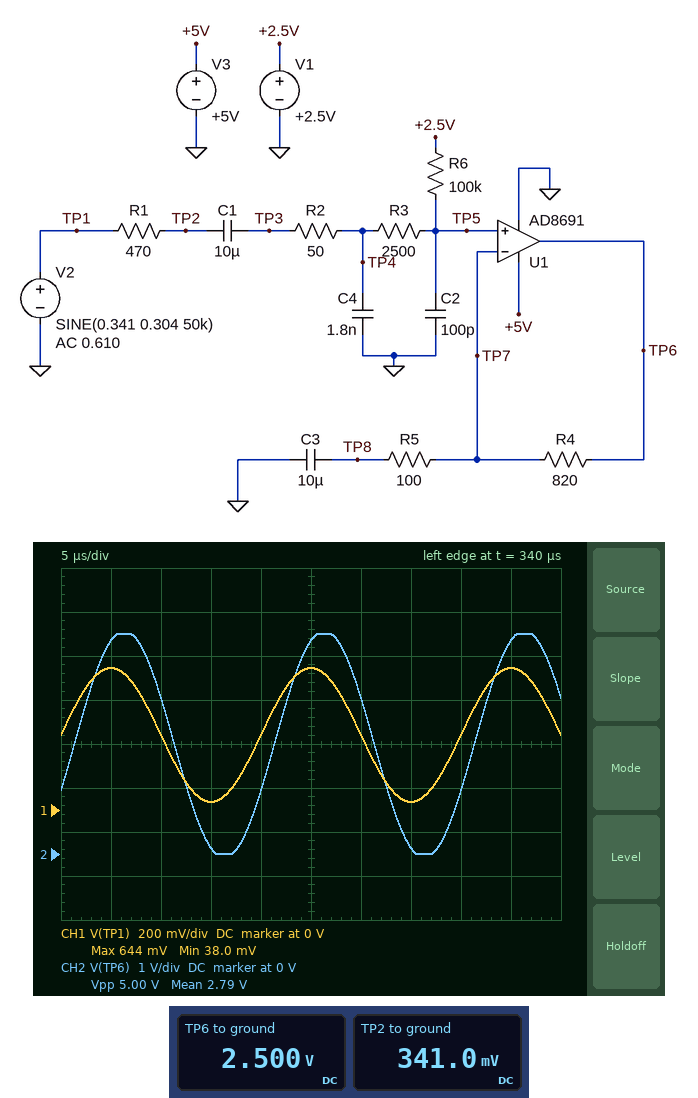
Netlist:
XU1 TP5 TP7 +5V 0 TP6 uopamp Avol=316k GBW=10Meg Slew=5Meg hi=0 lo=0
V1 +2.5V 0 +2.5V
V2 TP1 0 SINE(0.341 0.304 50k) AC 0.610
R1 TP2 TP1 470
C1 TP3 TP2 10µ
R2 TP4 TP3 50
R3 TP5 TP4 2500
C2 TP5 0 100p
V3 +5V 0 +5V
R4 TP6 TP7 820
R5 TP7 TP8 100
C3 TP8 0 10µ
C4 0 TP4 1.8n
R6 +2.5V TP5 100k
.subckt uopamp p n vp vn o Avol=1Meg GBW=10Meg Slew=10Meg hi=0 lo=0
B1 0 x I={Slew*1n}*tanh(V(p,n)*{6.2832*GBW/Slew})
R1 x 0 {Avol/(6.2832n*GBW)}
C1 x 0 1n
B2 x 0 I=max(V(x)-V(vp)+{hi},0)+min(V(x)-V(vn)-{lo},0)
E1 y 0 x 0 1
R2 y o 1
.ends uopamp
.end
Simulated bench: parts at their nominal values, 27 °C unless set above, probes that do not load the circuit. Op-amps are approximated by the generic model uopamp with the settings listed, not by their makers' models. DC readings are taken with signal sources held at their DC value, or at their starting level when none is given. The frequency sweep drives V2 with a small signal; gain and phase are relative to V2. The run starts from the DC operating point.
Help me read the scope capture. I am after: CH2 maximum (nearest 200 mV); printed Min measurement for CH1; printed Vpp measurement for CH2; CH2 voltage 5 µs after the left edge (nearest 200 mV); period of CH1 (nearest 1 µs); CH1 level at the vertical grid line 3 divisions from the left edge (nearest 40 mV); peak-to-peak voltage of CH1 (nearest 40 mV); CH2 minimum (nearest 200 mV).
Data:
5.0 V
38.0 mV
5.00 V
4.8 V
20 µs
40 mV
600 mV
0 V
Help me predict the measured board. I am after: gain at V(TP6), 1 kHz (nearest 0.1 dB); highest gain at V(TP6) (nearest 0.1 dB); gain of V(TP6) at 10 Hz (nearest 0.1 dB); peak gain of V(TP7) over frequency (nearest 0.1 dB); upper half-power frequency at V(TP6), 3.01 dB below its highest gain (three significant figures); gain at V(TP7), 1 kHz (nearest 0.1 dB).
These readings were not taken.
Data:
18.9 dB
19.0 dB
1.0 dB
-0.3 dB
150 kHz
-0.3 dB
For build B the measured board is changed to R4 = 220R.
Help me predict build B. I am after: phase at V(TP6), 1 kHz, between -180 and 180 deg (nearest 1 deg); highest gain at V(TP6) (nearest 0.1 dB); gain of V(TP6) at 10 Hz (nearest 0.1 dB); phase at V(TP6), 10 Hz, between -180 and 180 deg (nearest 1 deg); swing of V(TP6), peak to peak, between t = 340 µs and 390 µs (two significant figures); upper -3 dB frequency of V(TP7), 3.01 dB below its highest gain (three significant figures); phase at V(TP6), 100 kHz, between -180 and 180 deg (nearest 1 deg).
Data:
6 deg
9.8 dB
-0.1 dB
9 deg
1.8 V
152 kHz
-42 deg
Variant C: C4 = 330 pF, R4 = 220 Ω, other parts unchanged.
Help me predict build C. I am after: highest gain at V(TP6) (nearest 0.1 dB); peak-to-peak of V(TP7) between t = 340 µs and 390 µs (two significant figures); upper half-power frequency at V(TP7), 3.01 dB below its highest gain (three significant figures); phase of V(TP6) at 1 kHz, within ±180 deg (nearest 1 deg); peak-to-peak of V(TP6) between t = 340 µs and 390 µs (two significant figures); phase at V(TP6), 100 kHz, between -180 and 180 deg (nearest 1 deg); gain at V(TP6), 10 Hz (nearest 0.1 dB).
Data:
9.8 dB
590 mV
413 kHz
6 deg
1.9 V
-18 deg
-0.1 dB
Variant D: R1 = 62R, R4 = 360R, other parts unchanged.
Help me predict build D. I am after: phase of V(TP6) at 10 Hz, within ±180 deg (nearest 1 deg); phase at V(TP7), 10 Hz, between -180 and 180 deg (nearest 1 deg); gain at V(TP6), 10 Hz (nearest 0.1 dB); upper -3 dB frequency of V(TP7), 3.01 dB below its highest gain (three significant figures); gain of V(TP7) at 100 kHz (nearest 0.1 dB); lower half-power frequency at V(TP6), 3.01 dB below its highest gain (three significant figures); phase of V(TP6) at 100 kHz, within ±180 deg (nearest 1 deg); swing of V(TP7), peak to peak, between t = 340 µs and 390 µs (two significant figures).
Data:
13 deg
1 deg
0.1 dB
429 kHz
-0.4 dB
151 Hz
-19 deg
590 mV
